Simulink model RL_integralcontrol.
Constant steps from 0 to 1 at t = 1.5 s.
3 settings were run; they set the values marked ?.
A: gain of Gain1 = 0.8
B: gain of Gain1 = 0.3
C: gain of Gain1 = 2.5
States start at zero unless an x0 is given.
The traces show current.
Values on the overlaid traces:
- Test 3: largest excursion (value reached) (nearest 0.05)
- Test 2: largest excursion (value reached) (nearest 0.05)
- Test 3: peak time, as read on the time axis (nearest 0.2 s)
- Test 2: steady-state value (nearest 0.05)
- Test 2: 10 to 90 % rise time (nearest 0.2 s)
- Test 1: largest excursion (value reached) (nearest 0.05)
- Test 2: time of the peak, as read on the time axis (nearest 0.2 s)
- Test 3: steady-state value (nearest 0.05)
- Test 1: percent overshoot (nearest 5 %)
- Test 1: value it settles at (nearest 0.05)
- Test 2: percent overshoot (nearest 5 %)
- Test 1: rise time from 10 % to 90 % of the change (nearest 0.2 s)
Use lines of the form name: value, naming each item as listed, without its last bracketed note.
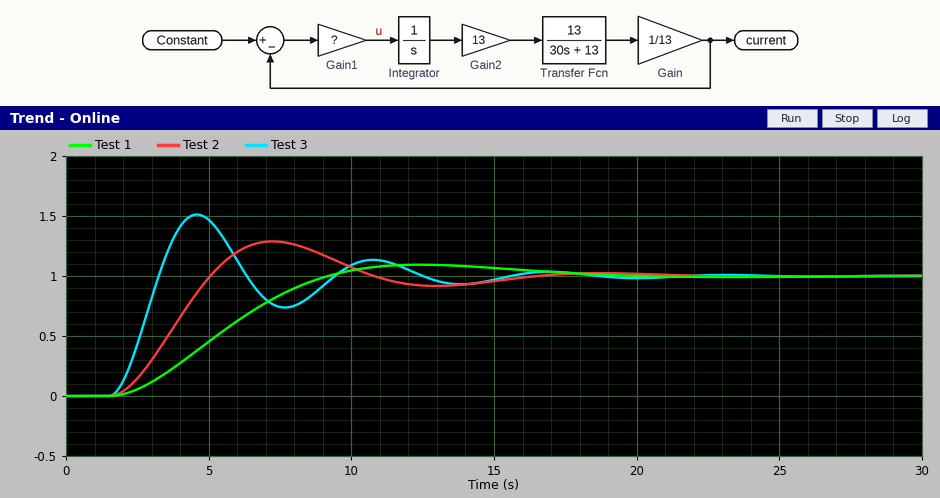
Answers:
Test 3: largest excursion (value reached): 1.50
Test 2: largest excursion (value reached): 1.30
Test 3: peak time, as read on the time axis: 4.6 s
Test 2: steady-state value: 1.00
Test 2: 10 to 90 % rise time: 2.4 s
Test 1: largest excursion (value reached): 1.10
Test 2: time of the peak, as read on the time axis: 7.2 s
Test 3: steady-state value: 1.00
Test 1: percent overshoot: 10 %
Test 1: value it settles at: 1.00
Test 2: percent overshoot: 30 %
Test 1: rise time from 10 % to 90 % of the change: 5.2 s
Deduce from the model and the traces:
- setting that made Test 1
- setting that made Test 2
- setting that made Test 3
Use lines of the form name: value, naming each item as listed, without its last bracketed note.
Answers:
setting that made Test 1: B
setting that made Test 2: A
setting that made Test 3: C
